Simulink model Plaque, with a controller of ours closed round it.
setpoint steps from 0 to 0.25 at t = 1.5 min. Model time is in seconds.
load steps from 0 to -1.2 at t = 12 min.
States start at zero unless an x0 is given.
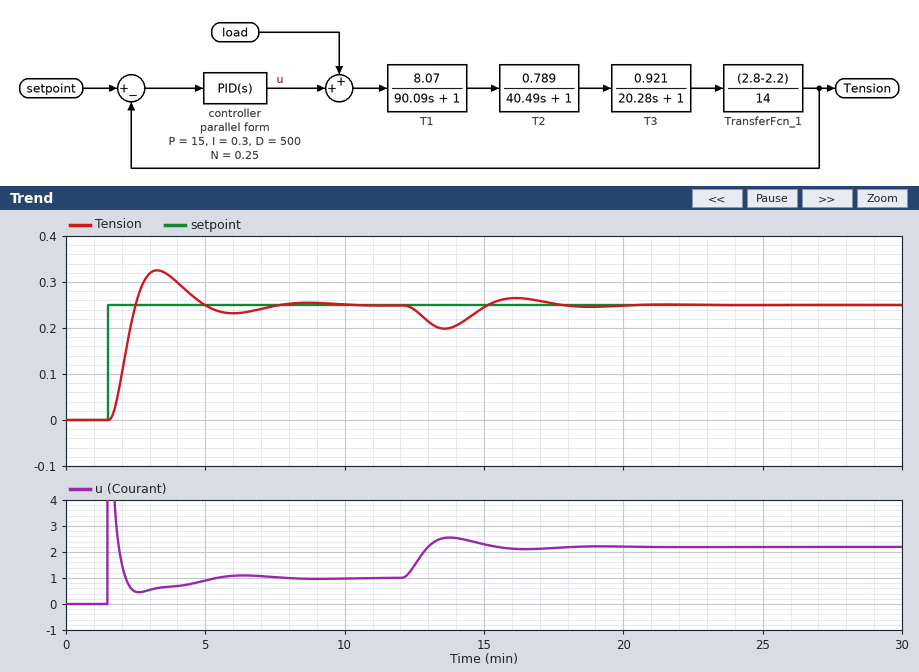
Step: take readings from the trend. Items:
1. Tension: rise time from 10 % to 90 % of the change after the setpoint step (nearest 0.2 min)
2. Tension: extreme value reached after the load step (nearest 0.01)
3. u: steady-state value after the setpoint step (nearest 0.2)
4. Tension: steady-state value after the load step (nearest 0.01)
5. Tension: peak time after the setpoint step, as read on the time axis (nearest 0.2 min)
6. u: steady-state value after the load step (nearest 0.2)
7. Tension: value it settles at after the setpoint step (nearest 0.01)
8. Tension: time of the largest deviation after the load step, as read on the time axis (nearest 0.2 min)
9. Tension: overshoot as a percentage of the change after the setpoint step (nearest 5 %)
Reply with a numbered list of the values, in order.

1. 0.6 min
2. 0.20
3. 1.0
4. 0.25
5. 3.2 min
6. 2.2
7. 0.25
8. 13.6 min
9. 30 %
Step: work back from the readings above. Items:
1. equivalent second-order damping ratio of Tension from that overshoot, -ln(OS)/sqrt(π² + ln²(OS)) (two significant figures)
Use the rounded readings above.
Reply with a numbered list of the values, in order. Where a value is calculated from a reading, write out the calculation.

1. ln(0.3) = -1.204; 1.204 / sqrt(9.870 + 1.450) = 0.36
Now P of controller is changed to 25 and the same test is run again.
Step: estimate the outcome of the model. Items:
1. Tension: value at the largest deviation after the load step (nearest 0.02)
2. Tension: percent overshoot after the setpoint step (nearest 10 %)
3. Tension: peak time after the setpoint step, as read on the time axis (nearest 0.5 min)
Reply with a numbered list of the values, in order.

1. 0.20
2. 40 %
3. 3.0 min
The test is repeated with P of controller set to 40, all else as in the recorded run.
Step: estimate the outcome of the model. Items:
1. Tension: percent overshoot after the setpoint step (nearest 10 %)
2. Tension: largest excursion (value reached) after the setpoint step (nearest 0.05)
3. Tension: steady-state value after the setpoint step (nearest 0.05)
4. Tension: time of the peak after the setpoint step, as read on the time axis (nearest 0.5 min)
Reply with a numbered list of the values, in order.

1. 60 %
2. 0.40
3. 0.25
4. 2.5 min
